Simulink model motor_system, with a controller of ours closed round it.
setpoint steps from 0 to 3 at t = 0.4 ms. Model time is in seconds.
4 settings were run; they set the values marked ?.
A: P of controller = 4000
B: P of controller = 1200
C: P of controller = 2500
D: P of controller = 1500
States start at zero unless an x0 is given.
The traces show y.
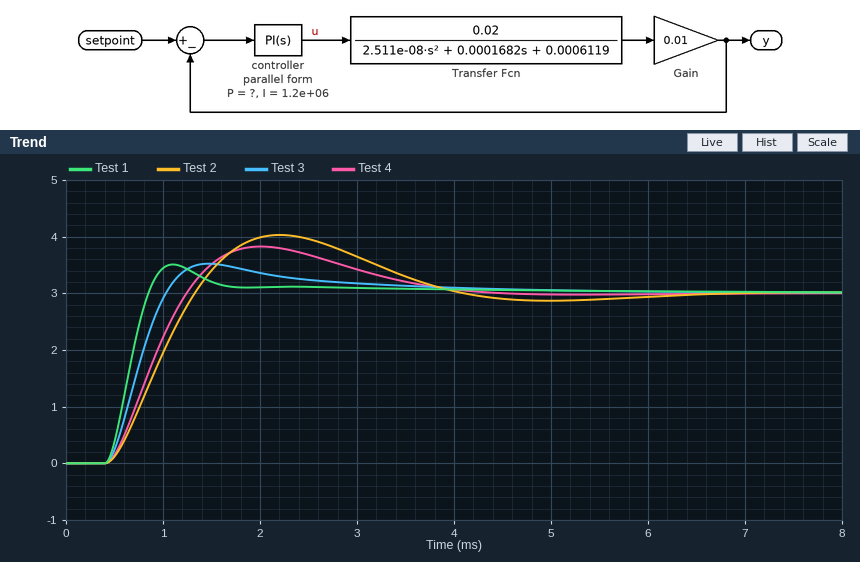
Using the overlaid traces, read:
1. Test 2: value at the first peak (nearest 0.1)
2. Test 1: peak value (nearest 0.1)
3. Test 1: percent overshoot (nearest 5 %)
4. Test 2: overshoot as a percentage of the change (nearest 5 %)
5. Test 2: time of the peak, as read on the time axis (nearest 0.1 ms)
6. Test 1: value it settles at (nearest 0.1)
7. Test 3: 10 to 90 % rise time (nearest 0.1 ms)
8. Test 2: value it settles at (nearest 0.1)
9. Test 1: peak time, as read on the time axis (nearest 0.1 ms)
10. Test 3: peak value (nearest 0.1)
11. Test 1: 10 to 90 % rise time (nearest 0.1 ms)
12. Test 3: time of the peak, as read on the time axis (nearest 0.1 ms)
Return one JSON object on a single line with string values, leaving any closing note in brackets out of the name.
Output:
{"Test 2: value at the first peak": "4.0", "Test 1: peak value": "3.5", "Test 1: percent overshoot": "15 %", "Test 2: overshoot as a percentage of the change": "35 %", "Test 2: time of the peak, as read on the time axis": "2.2 ms", "Test 1: value it settles at": "3.0", "Test 3: 10 to 90 % rise time": "0.4 ms", "Test 2: value it settles at": "3.0", "Test 1: peak time, as read on the time axis": "1.1 ms", "Test 3: peak value": "3.5", "Test 1: 10 to 90 % rise time": "0.3 ms", "Test 3: time of the peak, as read on the time axis": "1.5 ms"}
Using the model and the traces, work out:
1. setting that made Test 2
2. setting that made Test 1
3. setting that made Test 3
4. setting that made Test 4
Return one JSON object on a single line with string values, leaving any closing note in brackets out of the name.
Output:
{"setting that made Test 2": "B", "setting that made Test 1": "A", "setting that made Test 3": "C", "setting that made Test 4": "D"}
